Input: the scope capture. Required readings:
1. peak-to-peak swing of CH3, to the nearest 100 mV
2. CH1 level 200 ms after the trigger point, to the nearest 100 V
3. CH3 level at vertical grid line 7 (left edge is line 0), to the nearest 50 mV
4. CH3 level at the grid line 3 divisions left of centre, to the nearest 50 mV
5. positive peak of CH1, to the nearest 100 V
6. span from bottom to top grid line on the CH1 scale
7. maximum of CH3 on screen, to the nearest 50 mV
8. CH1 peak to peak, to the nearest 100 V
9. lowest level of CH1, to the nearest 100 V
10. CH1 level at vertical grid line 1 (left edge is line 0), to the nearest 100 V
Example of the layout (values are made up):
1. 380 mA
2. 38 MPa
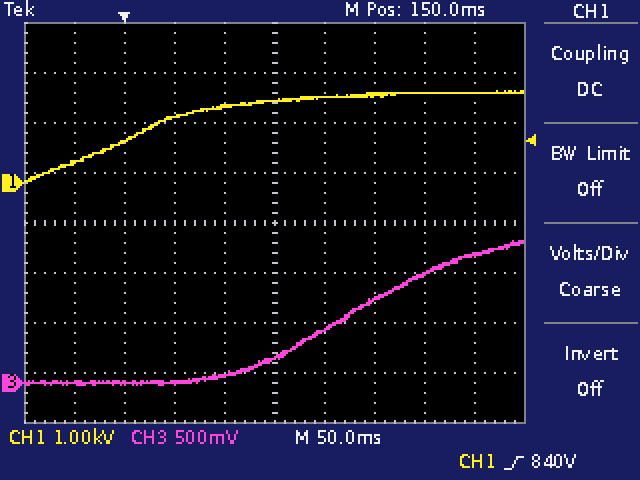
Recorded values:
1. 1.40 V
2. 1.7 kV
3. 850 mV
4. 0 mV
5. 1.8 kV
6. 8 kV
7. 1.40 V
8. 1.8 kV
9. 0.0 kV
10. 400 V
